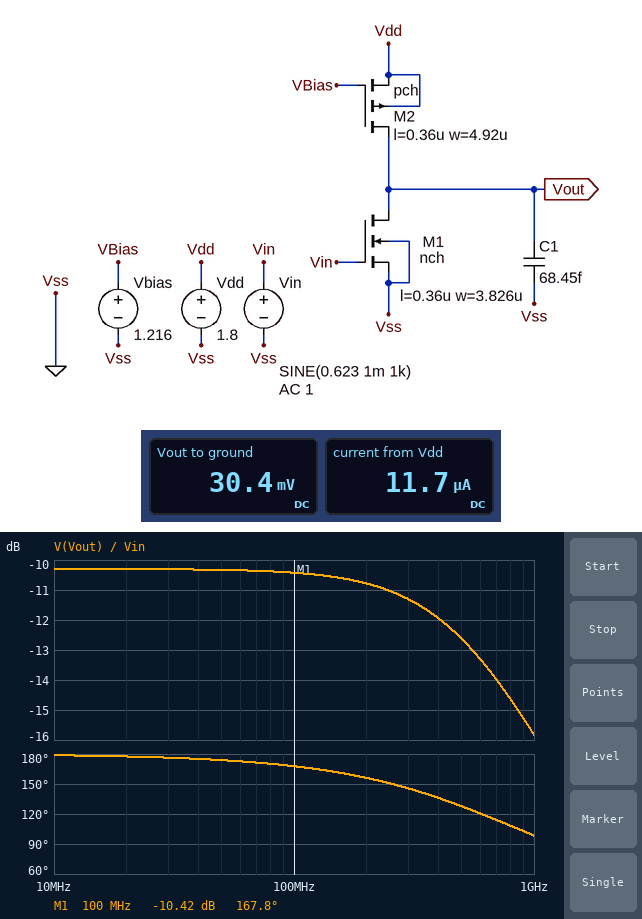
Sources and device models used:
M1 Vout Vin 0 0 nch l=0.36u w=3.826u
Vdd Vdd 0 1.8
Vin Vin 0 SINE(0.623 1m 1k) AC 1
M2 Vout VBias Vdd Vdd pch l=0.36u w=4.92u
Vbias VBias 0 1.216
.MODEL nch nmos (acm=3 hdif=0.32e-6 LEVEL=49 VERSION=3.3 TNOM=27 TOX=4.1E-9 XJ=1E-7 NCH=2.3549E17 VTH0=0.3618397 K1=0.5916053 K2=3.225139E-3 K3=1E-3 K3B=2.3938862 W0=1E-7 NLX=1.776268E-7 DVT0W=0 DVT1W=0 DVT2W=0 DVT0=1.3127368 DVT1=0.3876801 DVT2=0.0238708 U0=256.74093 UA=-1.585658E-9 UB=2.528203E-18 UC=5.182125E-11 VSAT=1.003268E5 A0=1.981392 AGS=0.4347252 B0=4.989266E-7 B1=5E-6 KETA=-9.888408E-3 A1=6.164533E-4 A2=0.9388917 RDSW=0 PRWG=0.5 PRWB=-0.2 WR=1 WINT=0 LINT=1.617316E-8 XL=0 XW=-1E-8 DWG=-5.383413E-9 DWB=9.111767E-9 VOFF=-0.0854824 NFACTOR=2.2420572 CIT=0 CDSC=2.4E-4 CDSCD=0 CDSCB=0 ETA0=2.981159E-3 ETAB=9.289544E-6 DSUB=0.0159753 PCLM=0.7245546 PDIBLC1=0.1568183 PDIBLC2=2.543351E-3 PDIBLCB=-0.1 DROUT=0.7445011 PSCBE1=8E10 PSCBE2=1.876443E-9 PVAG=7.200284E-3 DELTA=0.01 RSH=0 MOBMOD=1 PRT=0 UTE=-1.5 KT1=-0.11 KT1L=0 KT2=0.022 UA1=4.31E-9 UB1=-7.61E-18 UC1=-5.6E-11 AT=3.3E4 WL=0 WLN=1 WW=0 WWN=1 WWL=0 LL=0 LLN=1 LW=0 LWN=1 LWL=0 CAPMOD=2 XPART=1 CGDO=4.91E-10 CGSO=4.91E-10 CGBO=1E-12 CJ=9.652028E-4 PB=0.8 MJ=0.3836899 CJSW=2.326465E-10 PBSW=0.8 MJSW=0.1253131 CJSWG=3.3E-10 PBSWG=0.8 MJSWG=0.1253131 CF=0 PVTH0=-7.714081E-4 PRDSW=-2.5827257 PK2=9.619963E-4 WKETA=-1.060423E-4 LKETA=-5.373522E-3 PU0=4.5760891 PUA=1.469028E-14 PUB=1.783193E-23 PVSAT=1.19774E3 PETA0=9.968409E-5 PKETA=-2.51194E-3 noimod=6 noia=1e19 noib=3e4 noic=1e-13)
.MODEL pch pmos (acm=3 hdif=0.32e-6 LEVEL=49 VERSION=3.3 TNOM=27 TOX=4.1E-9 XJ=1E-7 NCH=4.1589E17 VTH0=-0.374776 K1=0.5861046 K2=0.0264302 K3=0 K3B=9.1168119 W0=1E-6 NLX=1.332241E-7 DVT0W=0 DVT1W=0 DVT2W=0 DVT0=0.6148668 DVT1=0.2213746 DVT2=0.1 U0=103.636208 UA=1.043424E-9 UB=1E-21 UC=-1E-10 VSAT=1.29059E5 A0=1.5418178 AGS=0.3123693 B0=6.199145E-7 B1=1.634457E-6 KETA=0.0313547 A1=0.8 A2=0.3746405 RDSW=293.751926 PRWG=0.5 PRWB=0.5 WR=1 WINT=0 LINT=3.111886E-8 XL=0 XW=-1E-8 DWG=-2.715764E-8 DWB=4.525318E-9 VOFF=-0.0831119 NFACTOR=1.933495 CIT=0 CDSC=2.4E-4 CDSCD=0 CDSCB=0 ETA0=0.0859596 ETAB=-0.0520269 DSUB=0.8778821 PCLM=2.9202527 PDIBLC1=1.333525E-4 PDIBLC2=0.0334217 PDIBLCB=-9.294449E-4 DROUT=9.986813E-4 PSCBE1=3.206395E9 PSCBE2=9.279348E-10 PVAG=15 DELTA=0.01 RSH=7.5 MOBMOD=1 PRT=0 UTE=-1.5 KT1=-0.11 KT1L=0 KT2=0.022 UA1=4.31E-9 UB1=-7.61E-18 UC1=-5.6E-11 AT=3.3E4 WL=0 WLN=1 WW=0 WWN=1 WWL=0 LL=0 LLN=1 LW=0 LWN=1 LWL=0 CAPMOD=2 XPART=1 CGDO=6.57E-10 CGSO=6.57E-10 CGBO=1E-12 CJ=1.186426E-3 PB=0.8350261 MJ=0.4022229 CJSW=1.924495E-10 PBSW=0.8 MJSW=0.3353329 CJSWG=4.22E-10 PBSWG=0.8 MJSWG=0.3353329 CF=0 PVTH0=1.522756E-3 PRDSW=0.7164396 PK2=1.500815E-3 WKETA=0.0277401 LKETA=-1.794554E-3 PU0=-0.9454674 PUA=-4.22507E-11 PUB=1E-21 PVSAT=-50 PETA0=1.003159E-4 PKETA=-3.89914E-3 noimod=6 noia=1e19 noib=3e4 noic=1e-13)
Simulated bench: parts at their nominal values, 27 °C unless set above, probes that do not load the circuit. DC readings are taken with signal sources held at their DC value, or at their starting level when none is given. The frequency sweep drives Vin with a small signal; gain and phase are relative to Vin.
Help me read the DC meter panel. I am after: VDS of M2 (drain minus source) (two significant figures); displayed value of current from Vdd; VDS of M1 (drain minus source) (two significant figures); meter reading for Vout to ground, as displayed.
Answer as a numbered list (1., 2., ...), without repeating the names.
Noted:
1. -1.8 V
2. 11.7 µA
3. 30 mV
4. 30.4 mV
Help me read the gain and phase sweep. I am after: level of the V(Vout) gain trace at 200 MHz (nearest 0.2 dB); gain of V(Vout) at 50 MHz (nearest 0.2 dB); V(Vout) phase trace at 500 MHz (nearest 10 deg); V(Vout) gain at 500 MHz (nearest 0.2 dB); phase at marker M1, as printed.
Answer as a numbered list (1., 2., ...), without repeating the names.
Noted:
1. -10.8 dB
2. -10.4 dB
3. 130 deg
4. -12.6 dB
5. 167.8 deg
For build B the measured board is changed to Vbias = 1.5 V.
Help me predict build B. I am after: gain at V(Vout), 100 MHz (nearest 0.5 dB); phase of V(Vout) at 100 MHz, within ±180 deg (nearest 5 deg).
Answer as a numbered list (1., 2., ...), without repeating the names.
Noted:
1. -40.0 dB
2. 85 deg
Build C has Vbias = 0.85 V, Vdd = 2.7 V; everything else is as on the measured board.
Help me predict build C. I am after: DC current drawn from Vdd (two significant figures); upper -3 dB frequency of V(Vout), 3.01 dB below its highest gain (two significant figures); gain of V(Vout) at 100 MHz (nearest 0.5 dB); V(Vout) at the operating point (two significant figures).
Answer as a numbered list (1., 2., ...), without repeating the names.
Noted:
1. 45 µA
2. 1.7 GHz
3. -7.0 dB
4. 2.7 V
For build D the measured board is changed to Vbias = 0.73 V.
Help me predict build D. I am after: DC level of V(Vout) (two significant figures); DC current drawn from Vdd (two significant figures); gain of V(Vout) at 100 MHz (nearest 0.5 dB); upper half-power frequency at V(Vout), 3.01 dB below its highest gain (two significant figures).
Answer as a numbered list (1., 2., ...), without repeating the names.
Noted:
1. 1.7 V
2. 40 µA
3. -1.0 dB
4. 830 MHz
